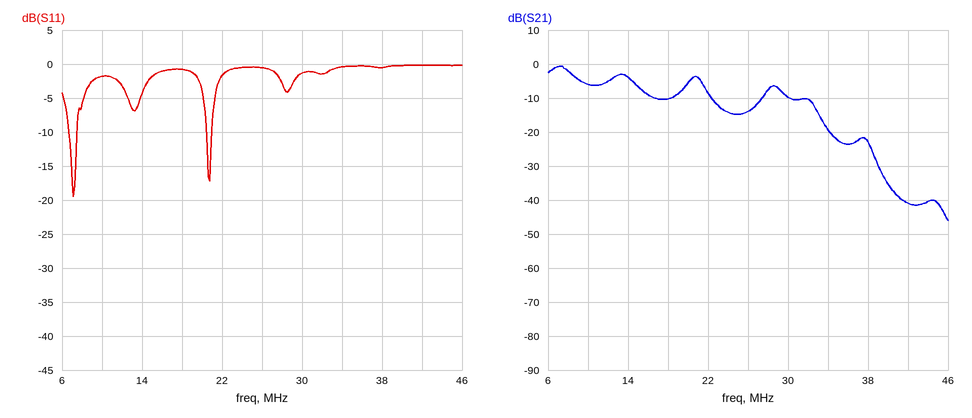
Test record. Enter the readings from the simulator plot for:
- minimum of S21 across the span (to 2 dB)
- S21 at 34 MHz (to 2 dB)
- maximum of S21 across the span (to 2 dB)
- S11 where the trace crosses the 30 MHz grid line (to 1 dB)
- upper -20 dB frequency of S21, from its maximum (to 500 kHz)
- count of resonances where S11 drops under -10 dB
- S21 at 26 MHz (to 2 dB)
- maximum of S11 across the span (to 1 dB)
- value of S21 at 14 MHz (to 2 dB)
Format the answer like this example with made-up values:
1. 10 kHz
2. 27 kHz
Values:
1. -46 dB
2. -20 dB
3. 0 dB
4. -1 dB
5. 34.5 MHz
6. 2
7. -14 dB
8. 0 dB
9. -4 dB
